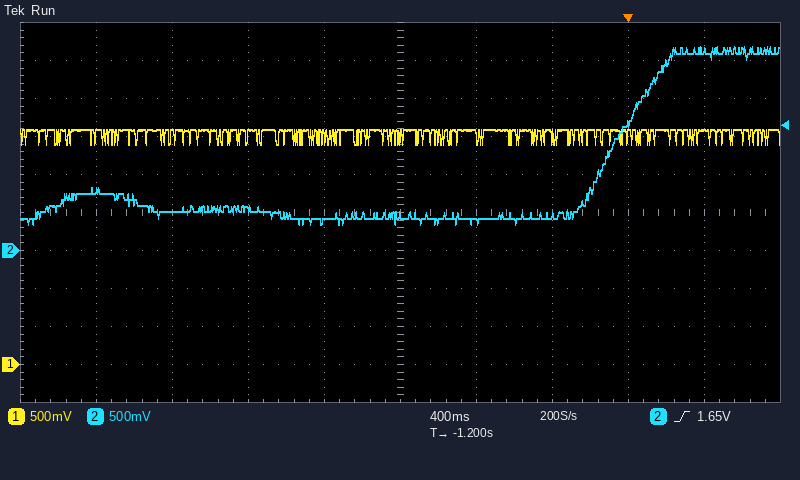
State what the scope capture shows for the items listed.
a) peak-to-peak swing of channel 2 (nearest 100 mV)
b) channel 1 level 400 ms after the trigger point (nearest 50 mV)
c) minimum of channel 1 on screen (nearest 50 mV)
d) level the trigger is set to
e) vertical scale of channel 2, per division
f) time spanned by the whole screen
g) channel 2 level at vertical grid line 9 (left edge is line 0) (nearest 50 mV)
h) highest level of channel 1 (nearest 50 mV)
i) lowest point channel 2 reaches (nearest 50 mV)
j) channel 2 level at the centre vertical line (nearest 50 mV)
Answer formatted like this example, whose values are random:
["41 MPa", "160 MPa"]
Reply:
["2.30 V", "3.10 V", "2.90 V", "1.65 V", "500 mV", "4 s", "2.65 V", "3.10 V", "350 mV", "450 mV"]
